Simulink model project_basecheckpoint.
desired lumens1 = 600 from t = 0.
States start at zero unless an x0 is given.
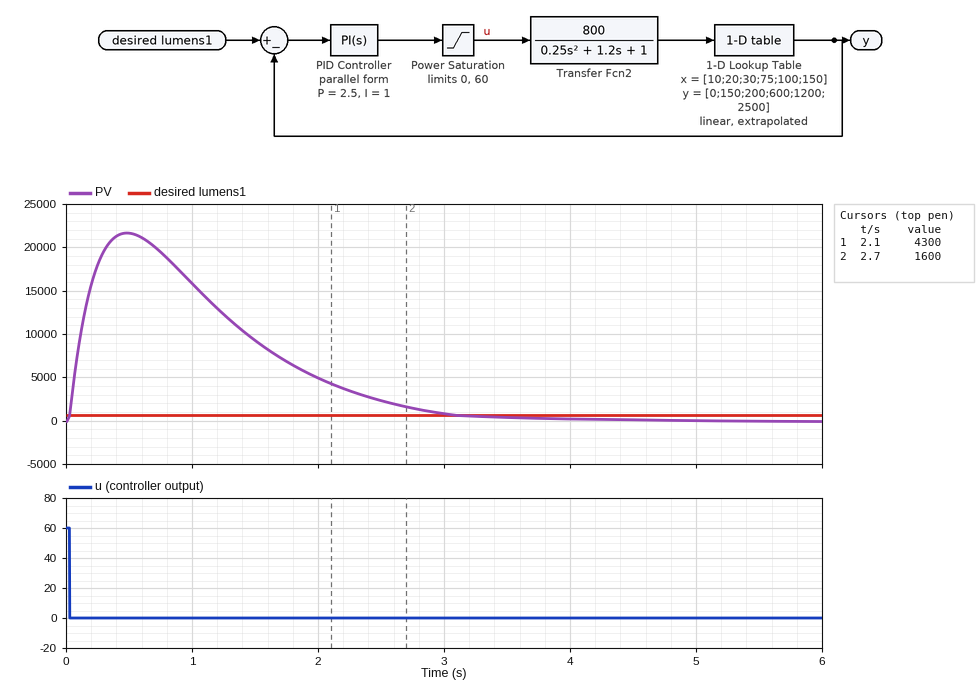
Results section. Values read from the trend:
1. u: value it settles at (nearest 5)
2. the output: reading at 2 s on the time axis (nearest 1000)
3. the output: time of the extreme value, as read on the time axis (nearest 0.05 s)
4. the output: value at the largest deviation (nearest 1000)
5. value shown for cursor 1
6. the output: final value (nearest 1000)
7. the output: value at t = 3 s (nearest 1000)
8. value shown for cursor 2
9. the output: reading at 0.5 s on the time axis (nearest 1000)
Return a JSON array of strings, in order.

["0", "5000", "0.50 s", "22000", "4300", "0", "1000", "1600", "22000"]
